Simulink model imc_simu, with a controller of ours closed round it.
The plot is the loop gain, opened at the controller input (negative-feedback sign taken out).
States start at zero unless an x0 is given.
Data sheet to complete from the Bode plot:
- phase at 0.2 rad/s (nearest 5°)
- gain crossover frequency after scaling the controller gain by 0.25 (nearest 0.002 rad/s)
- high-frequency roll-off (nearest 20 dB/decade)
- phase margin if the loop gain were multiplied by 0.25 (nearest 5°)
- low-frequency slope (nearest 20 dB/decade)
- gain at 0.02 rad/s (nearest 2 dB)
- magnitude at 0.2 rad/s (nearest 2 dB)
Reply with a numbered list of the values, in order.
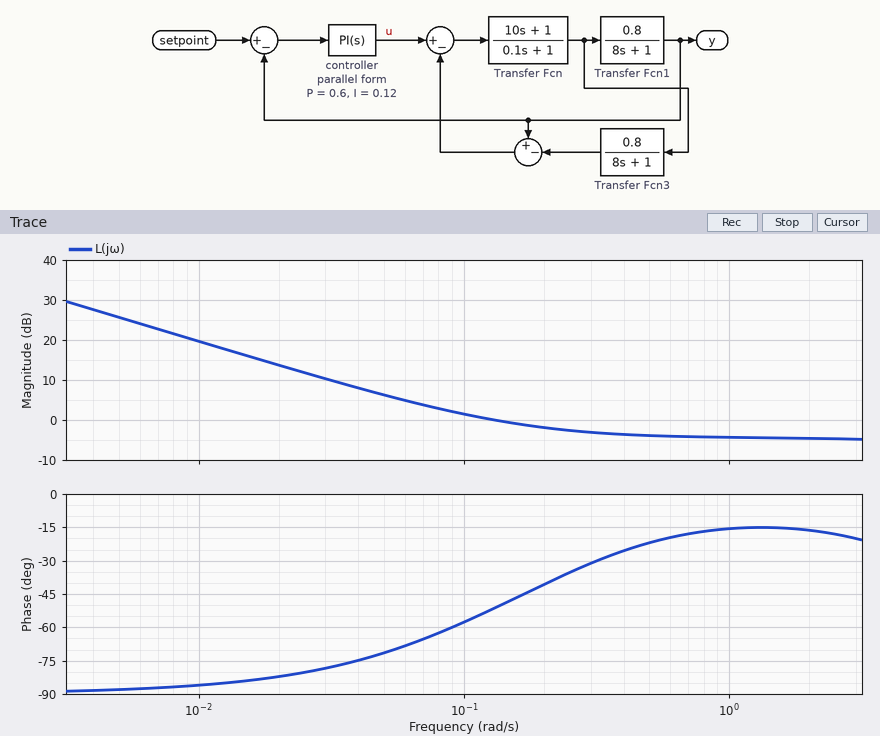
1. -40°
2. 0.024 rad/s
3. 0 dB/decade
4. 100°
5. -20 dB/decade
6. 14 dB
7. -2 dB
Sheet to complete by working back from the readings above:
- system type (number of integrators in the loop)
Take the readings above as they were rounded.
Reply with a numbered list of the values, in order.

1. 1
